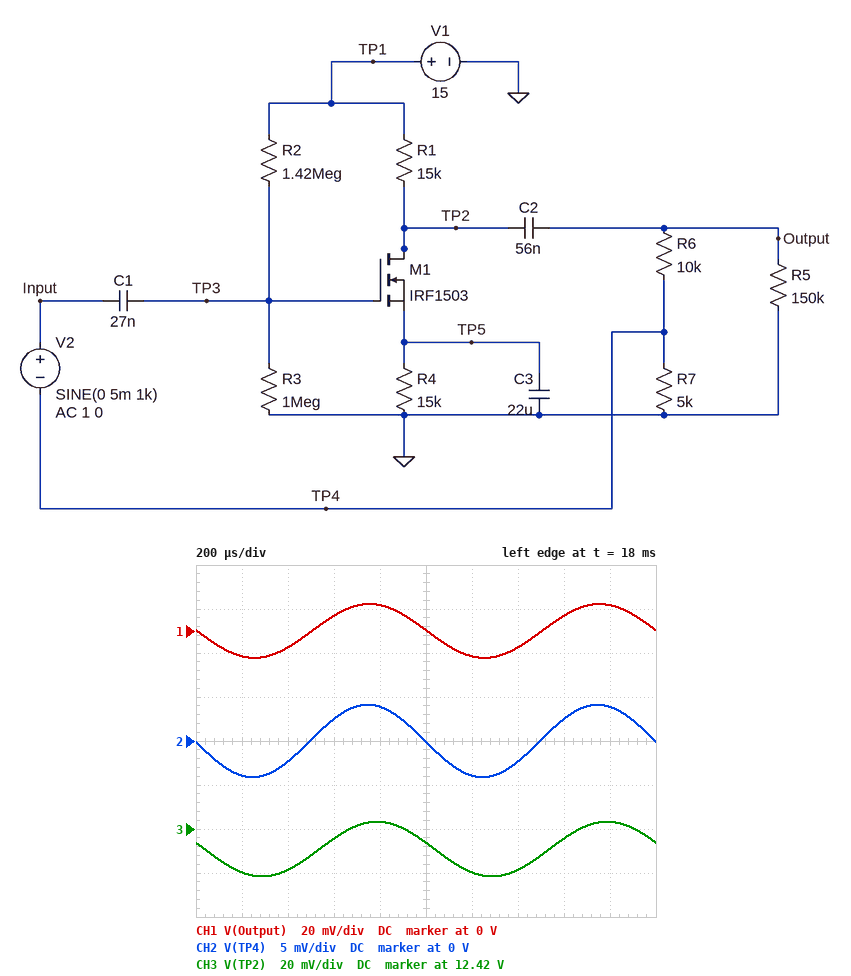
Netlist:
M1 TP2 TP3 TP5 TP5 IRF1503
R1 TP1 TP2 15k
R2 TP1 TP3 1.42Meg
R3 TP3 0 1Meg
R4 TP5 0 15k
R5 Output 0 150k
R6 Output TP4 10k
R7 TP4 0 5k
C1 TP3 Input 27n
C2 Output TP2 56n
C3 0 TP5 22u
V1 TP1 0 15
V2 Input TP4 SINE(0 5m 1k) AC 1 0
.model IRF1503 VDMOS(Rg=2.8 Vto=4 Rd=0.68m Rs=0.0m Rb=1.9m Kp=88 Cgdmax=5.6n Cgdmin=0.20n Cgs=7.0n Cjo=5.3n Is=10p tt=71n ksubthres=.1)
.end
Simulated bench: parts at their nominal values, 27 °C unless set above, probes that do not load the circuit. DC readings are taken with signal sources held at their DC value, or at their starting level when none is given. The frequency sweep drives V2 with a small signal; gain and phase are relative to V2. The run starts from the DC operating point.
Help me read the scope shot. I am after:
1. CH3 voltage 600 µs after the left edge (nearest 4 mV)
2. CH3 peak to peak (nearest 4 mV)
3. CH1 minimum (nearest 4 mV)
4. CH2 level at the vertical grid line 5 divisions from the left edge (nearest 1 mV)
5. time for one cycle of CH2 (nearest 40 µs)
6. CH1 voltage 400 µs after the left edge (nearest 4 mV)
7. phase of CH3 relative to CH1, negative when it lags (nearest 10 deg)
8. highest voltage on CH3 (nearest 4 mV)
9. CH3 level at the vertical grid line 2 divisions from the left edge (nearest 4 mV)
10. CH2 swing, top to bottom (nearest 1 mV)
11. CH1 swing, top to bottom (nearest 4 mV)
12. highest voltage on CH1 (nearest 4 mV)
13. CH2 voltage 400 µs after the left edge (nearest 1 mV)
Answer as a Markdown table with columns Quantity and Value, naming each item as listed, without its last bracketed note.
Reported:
| Quantity | Value |
|---|---|
| CH3 voltage 600 µs after the left edge | 12.416 V |
| CH3 peak to peak | 24 mV |
| CH1 minimum | -12 mV |
| CH2 level at the vertical grid line 5 divisions from the left edge | 0 V |
| time for one cycle of CH2 | 1.00 ms |
| CH1 voltage 400 µs after the left edge | -8 mV |
| phase of CH3 relative to CH1, negative when it lags | -10 deg |
| highest voltage on CH3 | 12.424 V |
| CH3 level at the vertical grid line 2 divisions from the left edge | 12.400 V |
| CH2 swing, top to bottom | 8 mV |
| CH1 swing, top to bottom | 24 mV |
| highest voltage on CH1 | 12 mV |
| CH2 voltage 400 µs after the left edge | -2 mV |
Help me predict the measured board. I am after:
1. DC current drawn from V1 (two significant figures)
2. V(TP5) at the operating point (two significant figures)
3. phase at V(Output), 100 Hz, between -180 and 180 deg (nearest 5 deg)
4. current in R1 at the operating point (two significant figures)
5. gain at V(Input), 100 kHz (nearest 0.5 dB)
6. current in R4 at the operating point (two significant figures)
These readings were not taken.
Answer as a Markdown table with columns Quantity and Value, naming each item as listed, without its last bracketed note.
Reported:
| Quantity | Value |
|---|---|
| DC current drawn from V1 | 180 µA |
| V(TP5) at the operating point | 2.6 V |
| phase at V(Output), 100 Hz, between -180 and 180 deg | -165 deg |
| current in R1 at the operating point | 170 µA |
| gain at V(Input), 100 kHz | -22.5 dB |
| current in R4 at the operating point | 170 µA |
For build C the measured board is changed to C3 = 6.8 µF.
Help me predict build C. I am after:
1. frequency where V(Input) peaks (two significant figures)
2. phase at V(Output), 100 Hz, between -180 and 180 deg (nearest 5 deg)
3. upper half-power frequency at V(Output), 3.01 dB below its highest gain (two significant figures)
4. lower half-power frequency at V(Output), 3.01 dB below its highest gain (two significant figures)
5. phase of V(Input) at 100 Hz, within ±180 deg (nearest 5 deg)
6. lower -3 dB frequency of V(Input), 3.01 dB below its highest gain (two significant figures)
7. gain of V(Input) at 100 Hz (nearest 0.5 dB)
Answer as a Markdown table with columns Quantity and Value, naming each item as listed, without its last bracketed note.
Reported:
| Quantity | Value |
|---|---|
| frequency where V(Input) peaks | 26 Hz |
| phase at V(Output), 100 Hz, between -180 and 180 deg | -160 deg |
| upper half-power frequency at V(Output), 3.01 dB below its highest gain | 16 kHz |
| lower half-power frequency at V(Output), 3.01 dB below its highest gain | 24 Hz |
| phase of V(Input) at 100 Hz, within ±180 deg | -55 deg |
| lower -3 dB frequency of V(Input), 3.01 dB below its highest gain | 12 Hz |
| gain of V(Input) at 100 Hz | -9.5 dB |
